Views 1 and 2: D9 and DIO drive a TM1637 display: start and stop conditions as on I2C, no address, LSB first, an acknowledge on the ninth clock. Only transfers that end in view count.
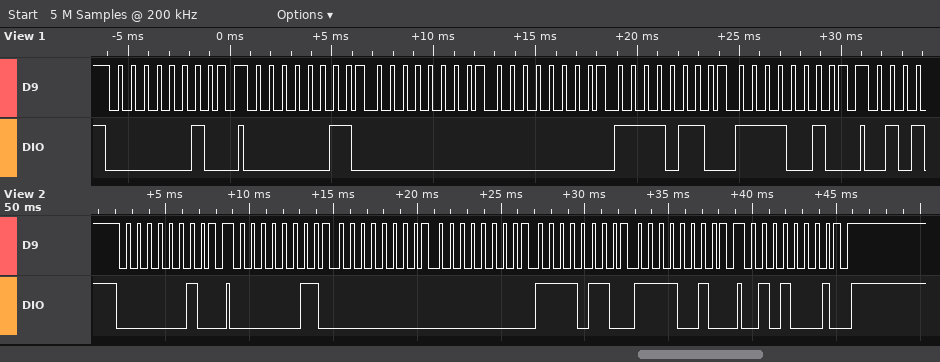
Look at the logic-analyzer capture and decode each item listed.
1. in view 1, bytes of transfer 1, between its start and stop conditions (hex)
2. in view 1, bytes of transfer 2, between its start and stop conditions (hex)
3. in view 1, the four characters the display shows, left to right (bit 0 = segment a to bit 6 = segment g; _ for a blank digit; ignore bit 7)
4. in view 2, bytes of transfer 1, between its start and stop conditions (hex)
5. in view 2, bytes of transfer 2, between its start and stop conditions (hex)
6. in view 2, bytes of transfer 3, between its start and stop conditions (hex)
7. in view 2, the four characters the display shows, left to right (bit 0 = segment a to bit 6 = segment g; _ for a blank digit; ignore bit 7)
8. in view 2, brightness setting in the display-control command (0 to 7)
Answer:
40
C0 00 00 6F 4F
__93
40
C0 00 00 6F 4F
8A
__93
2
